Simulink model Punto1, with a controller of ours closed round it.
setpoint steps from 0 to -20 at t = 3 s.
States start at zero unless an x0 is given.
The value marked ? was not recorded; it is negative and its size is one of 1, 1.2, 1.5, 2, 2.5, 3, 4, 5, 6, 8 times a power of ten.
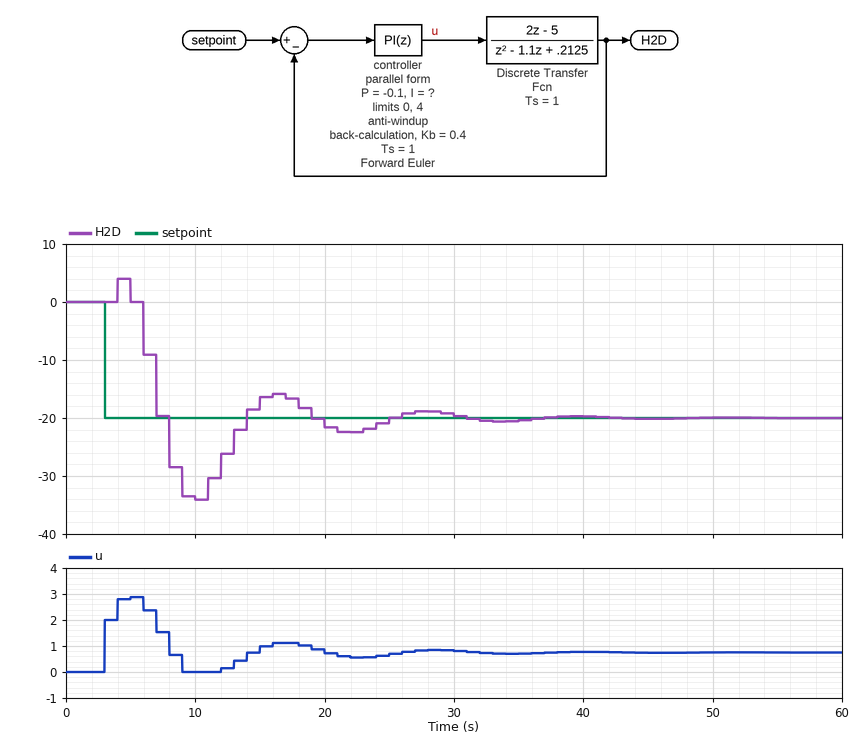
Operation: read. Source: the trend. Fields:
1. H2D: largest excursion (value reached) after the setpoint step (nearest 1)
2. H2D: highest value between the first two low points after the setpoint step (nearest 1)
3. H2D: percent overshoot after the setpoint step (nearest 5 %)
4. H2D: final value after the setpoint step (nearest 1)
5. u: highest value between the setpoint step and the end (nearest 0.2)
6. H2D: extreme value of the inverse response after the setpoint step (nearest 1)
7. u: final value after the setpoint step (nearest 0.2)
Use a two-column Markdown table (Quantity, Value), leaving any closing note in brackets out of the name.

| Quantity | Value |
|---|---|
| H2D: largest excursion (value reached) after the setpoint step | -34 |
| H2D: highest value between the first two low points after the setpoint step | -16 |
| H2D: percent overshoot after the setpoint step | 70 % |
| H2D: final value after the setpoint step | -20 |
| u: highest value between the setpoint step and the end | 2.8 |
| H2D: extreme value of the inverse response after the setpoint step | 4 |
| u: final value after the setpoint step | 0.8 |
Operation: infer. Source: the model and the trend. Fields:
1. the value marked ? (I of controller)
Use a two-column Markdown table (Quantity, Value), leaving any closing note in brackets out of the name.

| Quantity | Value |
|---|---|
| the value marked ? | -0.02 |
